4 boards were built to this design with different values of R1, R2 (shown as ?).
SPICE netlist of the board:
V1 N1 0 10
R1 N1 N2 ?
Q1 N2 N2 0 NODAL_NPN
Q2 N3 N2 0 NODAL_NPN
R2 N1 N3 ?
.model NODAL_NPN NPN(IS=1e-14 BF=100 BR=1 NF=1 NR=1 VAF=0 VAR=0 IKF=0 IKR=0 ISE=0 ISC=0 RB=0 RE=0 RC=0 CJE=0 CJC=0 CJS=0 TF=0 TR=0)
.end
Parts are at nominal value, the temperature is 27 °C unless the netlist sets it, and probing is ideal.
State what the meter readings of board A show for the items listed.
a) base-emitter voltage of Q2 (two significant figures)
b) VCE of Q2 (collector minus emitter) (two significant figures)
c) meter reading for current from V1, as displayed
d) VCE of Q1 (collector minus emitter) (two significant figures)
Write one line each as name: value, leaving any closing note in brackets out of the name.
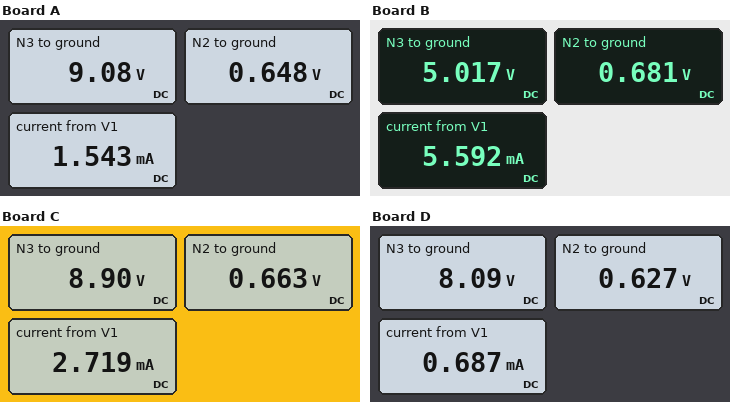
base-emitter voltage of Q2: 650 mV
VCE of Q2 (collector minus emitter): 9.1 V
meter reading for current from V1, as displayed: 1.543 mA
VCE of Q1 (collector minus emitter): 650 mV
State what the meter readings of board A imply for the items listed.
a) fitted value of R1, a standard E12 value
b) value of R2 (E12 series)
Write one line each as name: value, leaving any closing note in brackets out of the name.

fitted value of R1, a standard E12 value: 12 kΩ
value of R2: 1.2 kΩ
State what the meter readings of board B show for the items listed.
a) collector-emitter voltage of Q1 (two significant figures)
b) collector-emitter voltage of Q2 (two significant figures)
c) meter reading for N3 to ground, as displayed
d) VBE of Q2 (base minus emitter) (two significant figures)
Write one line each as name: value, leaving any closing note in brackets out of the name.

collector-emitter voltage of Q1: 680 mV
collector-emitter voltage of Q2: 5.0 V
meter reading for N3 to ground, as displayed: 5.017 V
VBE of Q2 (base minus emitter): 680 mV
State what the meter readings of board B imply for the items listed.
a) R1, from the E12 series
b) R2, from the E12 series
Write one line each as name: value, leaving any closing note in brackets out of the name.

R1, from the E12 series: 3.3 kΩ
R2, from the E12 series: 1.8 kΩ
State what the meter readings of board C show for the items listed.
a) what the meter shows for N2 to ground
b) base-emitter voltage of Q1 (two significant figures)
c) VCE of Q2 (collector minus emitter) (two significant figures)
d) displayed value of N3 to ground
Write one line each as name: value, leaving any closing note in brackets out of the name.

what the meter shows for N2 to ground: 0.663 V
base-emitter voltage of Q1: 660 mV
VCE of Q2 (collector minus emitter): 8.9 V
displayed value of N3 to ground: 8.90 V
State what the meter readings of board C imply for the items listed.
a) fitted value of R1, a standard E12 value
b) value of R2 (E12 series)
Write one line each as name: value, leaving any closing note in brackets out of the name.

fitted value of R1, a standard E12 value: 6.8 kΩ
value of R2: 820 Ω
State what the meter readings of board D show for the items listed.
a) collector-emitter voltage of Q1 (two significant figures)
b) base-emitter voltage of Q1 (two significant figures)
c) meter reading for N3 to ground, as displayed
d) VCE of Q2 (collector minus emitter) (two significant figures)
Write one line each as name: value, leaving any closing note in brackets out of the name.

collector-emitter voltage of Q1: 630 mV
base-emitter voltage of Q1: 630 mV
meter reading for N3 to ground, as displayed: 8.09 V
VCE of Q2 (collector minus emitter): 8.1 V
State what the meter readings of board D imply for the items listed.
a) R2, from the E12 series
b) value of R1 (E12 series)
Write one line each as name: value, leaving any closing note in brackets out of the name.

R2, from the E12 series: 5.6 kΩ
value of R1: 27 kΩ
